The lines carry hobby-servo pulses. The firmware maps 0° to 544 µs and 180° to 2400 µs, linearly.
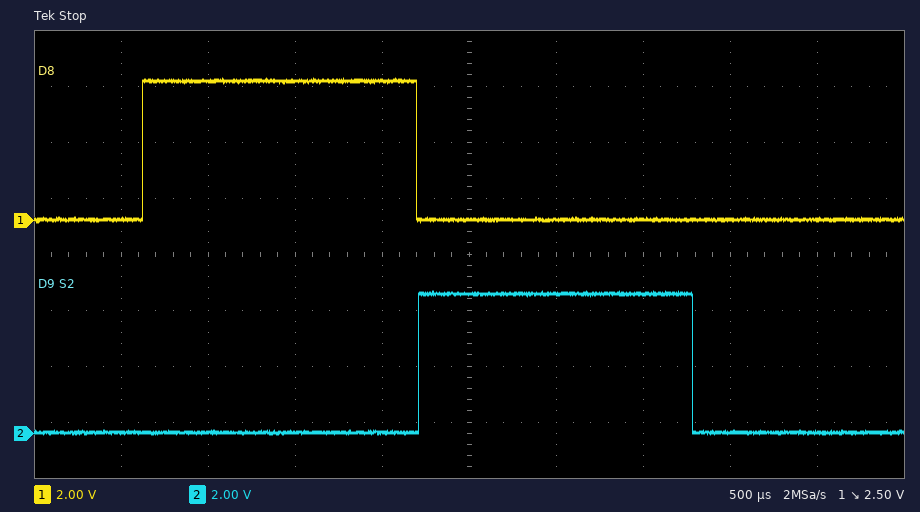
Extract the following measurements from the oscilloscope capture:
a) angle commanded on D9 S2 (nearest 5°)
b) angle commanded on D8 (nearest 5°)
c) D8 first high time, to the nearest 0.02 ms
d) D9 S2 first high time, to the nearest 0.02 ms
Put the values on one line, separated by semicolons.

100°; 100°; 1.58 ms; 1.58 ms
